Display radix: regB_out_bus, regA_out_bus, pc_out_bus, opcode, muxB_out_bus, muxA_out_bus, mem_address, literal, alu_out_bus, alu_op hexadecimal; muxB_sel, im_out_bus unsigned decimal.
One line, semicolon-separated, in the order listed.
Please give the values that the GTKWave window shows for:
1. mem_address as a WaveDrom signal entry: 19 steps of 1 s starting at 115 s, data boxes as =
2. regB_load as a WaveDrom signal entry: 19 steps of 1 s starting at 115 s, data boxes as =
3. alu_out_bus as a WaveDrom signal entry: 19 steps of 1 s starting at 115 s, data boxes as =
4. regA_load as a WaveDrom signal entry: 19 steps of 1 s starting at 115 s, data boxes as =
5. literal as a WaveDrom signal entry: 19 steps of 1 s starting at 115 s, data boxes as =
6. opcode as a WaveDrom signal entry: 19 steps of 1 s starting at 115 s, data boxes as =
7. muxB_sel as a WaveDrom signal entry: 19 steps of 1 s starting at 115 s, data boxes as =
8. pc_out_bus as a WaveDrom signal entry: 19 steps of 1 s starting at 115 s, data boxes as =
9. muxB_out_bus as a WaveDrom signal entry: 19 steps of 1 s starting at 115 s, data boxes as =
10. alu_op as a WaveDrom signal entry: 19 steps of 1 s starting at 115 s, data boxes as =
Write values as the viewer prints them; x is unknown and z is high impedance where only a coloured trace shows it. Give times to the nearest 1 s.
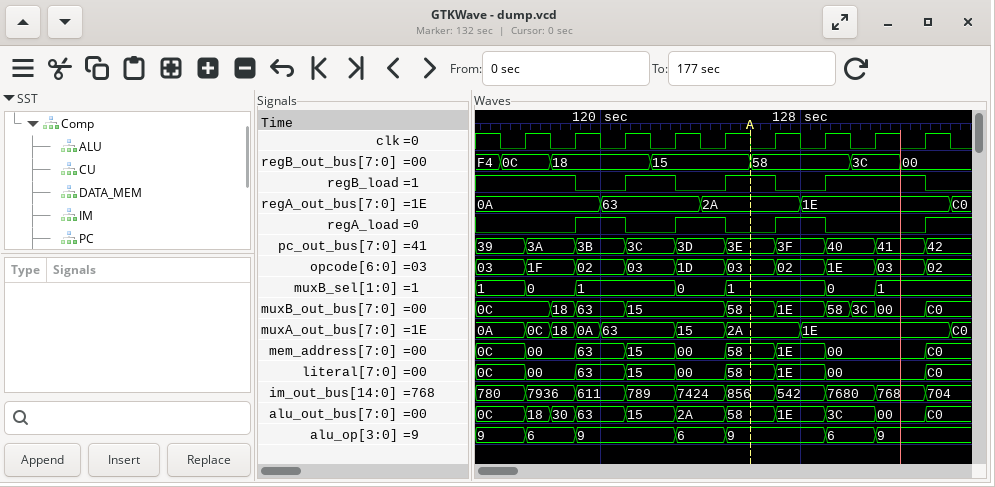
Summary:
{name: 'mem_address', wave: '=.=.=.=.=.=.=.=...=', data: '0C 00 63 15 00 58 1E 00 C0'}; {name: 'regB_load', wave: '1...0.1.0.1.0.1...0'}; {name: 'alu_out_bus', wave: '=.===.=.=.=.=.=.=.=', data: '0C 18 30 63 15 2A 58 1E 3C 00 C0'}; {name: 'regA_load', wave: '0...1.0.1.0.1.0...1'}; {name: 'literal', wave: '=.=.=.=.=.=.=.=...=', data: '0C 00 63 15 00 58 1E 00 C0'}; {name: 'opcode', wave: '=.=.=.=.=.=.=.=.=.=', data: '03 1F 02 03 1D 03 02 1E 03 02'}; {name: 'muxB_sel', wave: '=.=.=...=.=...=.=..', data: '1 0 1 0 1 0 1'}; {name: 'pc_out_bus', wave: '=.=.=.=.=.=.=.=.=.=', data: '39 3A 3B 3C 3D 3E 3F 40 41 42'}; {name: 'muxB_out_bus', wave: '=..==.=...=.=.===.=', data: '0C 18 63 15 58 1E 58 3C 00 C0'}; {name: 'alu_op', wave: '=.=.=...=.=...=.=..', data: '9 6 9 6 9 6 9'}
